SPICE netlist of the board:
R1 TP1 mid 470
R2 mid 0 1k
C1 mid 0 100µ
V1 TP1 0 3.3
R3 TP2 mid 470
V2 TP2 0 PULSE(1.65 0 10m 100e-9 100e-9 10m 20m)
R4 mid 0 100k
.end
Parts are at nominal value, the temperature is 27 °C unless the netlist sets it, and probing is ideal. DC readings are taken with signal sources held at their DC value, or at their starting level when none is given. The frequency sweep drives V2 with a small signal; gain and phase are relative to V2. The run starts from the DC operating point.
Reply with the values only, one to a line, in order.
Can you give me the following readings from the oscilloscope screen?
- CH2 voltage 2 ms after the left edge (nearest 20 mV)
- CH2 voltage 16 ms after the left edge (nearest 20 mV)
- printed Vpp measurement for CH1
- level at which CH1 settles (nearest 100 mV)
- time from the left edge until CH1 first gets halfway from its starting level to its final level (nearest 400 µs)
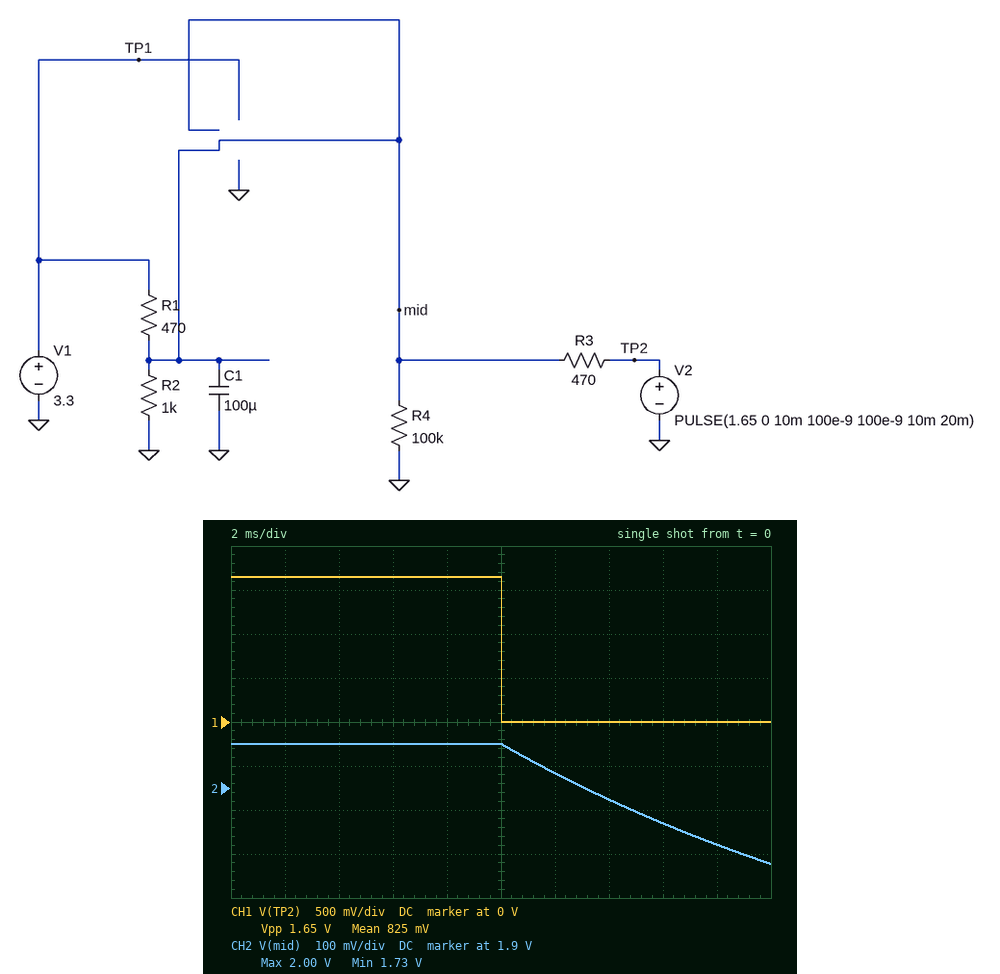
2.00 V
1.82 V
1.65 V
0 V
10.0 ms
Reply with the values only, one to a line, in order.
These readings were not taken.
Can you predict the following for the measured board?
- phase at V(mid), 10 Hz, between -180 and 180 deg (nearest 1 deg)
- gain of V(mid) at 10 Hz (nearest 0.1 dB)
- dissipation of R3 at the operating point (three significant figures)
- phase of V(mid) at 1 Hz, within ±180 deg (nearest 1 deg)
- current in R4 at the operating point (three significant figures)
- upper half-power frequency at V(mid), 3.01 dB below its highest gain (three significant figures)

-50 deg
-11.7 dB
261 µW
-7 deg
20.0 µA
8.38 Hz
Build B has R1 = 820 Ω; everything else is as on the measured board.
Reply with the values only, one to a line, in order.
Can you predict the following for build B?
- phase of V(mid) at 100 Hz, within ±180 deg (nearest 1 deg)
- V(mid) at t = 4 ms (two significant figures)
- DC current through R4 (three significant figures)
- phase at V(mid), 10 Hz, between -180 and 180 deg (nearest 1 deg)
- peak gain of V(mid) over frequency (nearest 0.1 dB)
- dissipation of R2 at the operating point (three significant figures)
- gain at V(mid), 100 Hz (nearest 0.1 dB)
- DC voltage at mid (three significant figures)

-86 deg
1.7 V
17.3 µA
-55 deg
-6.2 dB
2.99 mW
-29.4 dB
1.73 V
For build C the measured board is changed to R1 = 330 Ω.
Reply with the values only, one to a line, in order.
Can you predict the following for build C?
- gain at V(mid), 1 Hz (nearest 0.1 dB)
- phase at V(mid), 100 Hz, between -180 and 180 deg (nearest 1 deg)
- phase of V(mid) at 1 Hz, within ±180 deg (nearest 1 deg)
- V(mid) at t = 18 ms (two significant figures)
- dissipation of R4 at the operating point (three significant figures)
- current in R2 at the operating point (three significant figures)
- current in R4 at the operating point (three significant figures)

-9.3 dB
-84 deg
-6 deg
2.0 V
48.0 µW
2.19 mA
21.9 µA
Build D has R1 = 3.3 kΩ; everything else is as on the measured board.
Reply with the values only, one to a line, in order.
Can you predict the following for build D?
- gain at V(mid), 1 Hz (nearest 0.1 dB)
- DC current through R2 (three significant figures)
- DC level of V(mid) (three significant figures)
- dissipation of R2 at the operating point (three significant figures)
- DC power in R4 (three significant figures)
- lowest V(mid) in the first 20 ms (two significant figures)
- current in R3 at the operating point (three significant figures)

-4.3 dB
1.31 mA
1.31 V
1.72 mW
17.2 µW
1.0 V
721 µA
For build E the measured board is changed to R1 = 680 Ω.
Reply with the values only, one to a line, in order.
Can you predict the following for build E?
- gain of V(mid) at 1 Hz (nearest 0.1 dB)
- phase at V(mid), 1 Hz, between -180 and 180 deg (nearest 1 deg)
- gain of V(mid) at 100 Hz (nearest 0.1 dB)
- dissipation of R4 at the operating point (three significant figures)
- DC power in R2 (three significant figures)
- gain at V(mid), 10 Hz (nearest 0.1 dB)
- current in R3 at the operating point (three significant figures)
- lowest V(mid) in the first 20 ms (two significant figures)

-6.8 dB
-8 deg
-29.4 dB
32.9 µW
3.29 mW
-11.3 dB
351 µA
1.5 V
